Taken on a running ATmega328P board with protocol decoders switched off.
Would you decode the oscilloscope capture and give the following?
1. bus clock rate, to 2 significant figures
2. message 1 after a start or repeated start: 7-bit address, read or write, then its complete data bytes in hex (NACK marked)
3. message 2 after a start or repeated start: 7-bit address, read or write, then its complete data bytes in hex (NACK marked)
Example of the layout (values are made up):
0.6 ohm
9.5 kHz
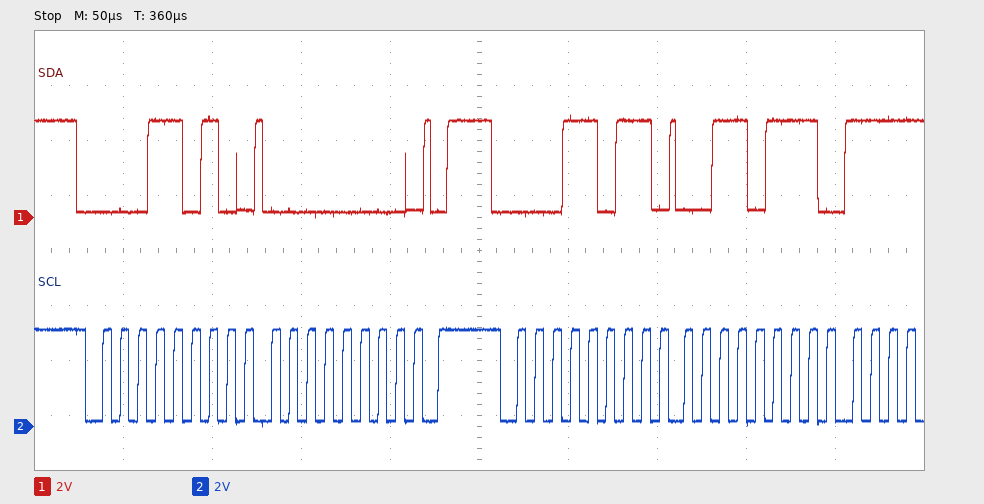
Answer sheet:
100 kHz
0x0D write: 00
0x0D read: 37
